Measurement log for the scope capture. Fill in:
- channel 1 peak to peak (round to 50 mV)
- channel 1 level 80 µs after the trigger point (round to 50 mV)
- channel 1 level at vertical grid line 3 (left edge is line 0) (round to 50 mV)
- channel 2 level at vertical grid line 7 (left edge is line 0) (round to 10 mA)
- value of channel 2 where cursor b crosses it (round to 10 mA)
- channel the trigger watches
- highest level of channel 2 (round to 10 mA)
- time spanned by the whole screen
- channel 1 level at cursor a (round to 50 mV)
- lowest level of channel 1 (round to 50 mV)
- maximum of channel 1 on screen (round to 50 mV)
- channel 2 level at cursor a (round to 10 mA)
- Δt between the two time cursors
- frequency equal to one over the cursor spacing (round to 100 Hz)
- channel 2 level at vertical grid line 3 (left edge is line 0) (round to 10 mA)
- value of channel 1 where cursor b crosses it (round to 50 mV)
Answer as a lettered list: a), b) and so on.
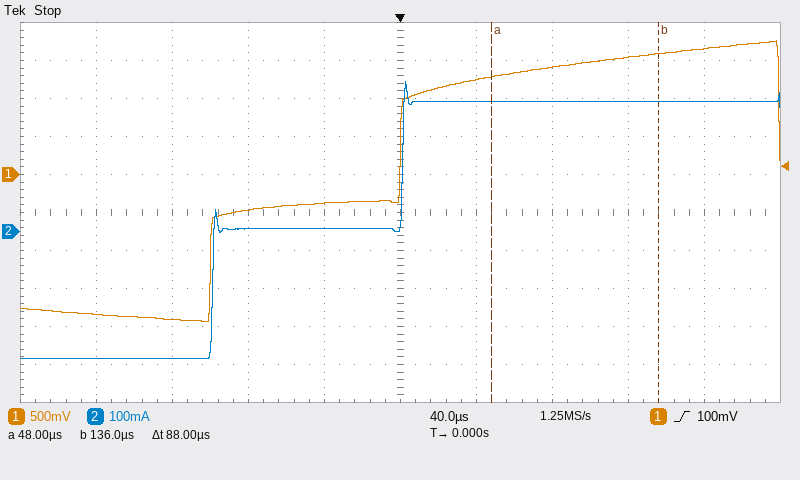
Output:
a) 3.70 V
b) 1.40 V
c) -450 mV
d) 340 mA
e) 340 mA
f) channel 1
g) 390 mA
h) 400 µs
i) 1.30 V
j) -1.95 V
k) 1.75 V
l) 340 mA
m) 88 µs
n) 11.4 kHz
o) 10 mA
p) 1.60 V
